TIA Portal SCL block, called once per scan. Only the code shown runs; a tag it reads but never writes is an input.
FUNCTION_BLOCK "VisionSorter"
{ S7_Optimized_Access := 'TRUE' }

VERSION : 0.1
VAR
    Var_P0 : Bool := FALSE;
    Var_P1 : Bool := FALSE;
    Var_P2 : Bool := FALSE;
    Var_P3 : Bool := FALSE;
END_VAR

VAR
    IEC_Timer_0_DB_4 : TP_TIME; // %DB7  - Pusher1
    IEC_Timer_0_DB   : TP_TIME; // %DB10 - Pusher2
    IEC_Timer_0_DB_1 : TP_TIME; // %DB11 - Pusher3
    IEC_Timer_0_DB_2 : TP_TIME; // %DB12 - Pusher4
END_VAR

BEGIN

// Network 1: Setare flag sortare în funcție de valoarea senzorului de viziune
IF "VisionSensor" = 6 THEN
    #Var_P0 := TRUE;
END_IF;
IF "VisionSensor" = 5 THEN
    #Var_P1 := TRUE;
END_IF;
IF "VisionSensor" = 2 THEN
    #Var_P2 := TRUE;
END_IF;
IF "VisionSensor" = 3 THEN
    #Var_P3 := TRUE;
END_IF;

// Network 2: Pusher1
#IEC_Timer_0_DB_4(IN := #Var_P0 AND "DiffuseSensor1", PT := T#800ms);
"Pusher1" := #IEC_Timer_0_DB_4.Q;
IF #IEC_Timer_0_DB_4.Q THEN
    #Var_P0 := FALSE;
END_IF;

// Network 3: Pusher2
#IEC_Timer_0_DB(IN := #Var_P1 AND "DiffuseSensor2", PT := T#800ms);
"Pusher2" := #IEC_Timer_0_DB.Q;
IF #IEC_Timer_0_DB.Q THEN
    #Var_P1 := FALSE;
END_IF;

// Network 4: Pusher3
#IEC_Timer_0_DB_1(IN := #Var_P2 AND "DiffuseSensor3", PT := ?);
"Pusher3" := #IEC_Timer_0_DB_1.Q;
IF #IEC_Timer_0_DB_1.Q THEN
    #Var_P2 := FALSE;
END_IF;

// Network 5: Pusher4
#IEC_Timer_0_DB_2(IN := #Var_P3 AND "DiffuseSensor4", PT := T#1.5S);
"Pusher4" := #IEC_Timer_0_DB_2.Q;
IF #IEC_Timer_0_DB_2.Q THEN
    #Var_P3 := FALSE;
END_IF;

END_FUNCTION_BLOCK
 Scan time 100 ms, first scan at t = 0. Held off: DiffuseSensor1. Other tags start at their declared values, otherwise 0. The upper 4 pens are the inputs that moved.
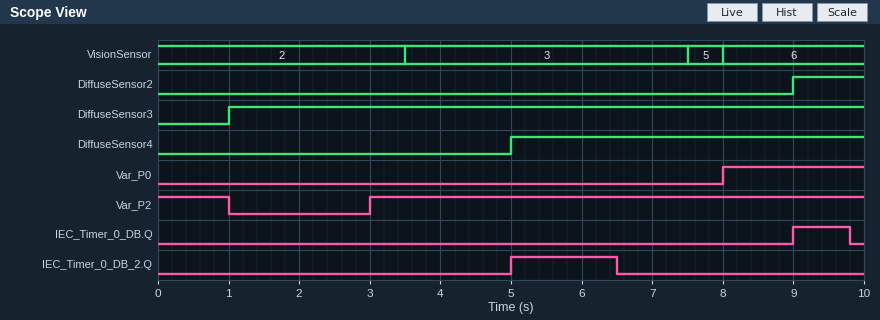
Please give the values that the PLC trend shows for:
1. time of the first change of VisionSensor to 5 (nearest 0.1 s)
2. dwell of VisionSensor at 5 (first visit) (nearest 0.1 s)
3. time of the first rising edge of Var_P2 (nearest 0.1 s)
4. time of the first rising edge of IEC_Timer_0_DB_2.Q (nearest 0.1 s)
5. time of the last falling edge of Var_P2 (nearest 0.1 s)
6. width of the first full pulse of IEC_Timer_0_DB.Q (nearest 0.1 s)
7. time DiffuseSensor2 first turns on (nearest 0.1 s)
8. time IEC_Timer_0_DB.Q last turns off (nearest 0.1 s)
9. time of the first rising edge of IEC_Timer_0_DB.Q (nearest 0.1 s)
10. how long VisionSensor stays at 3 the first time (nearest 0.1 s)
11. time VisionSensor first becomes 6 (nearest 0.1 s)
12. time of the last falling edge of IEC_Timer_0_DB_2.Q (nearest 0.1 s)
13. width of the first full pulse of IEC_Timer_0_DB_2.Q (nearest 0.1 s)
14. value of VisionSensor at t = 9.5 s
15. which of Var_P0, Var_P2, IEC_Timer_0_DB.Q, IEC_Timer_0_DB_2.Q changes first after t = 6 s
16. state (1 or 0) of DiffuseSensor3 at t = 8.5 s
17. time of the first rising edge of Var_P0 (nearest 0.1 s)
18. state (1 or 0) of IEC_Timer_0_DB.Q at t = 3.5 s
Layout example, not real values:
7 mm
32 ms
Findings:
7.5 s
0.5 s
3.0 s
5.0 s
1.0 s
0.8 s
9.0 s
9.8 s
9.0 s
4.0 s
8.0 s
6.5 s
1.5 s
6
IEC_Timer_0_DB_2.Q
1
8.0 s
0
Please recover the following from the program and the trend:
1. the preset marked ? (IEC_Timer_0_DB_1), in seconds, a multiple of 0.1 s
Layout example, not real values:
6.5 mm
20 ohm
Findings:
2.0 s
